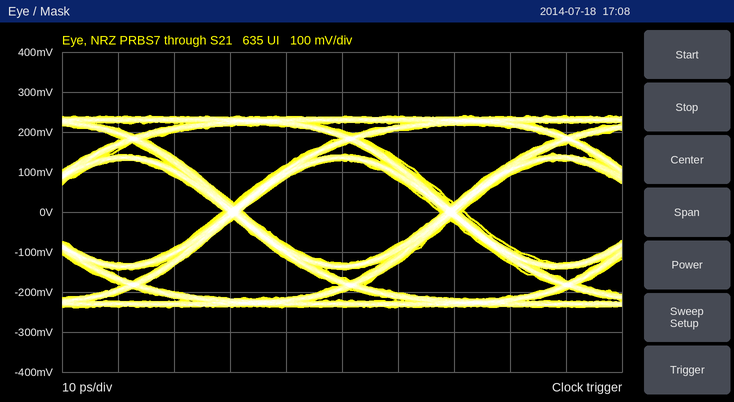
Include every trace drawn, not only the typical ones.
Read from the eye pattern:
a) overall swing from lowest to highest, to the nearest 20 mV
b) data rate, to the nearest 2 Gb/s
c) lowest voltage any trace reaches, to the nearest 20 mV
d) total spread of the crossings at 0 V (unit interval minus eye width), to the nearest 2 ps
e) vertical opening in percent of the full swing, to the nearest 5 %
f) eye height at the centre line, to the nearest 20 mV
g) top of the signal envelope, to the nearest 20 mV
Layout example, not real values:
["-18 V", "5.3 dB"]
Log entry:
["480 mV", "26 Gb/s", "-240 mV", "4 ps", "55 %", "260 mV", "240 mV"]
